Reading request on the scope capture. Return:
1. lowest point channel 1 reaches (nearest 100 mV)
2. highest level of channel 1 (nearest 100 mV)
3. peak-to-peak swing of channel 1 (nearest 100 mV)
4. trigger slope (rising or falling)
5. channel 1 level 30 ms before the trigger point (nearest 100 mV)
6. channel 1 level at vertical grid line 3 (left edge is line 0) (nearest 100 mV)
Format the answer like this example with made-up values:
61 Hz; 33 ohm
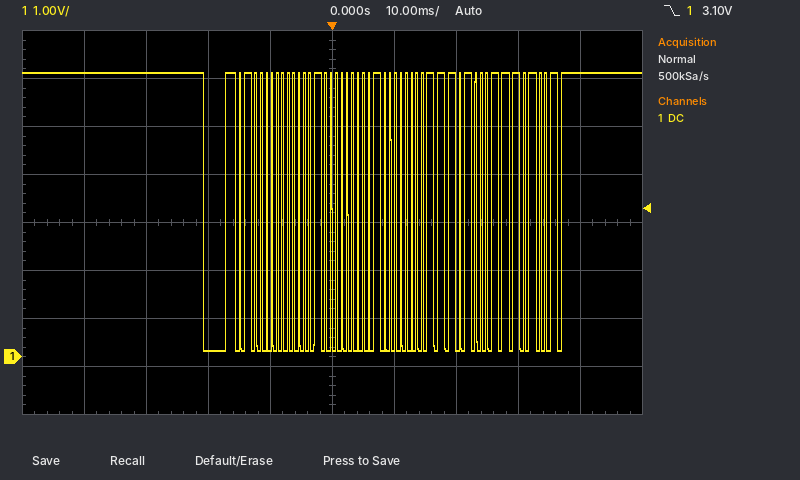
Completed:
100 mV; 5.9 V; 5.8 V; falling; 5.9 V; 100 mV
